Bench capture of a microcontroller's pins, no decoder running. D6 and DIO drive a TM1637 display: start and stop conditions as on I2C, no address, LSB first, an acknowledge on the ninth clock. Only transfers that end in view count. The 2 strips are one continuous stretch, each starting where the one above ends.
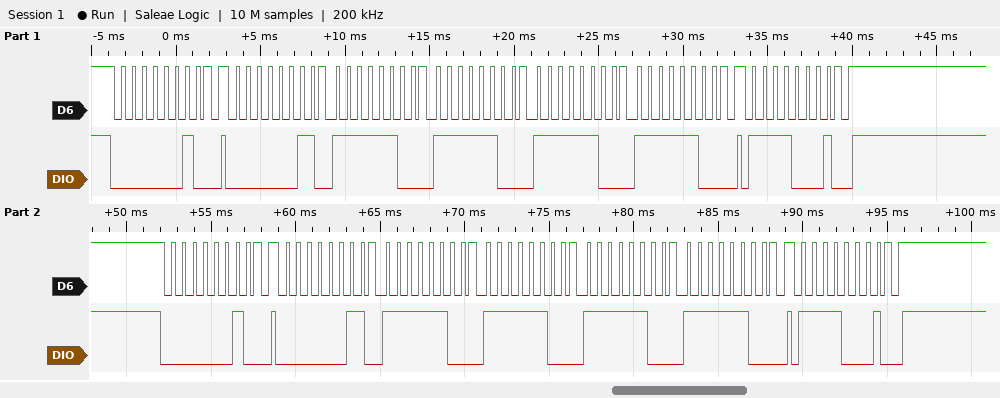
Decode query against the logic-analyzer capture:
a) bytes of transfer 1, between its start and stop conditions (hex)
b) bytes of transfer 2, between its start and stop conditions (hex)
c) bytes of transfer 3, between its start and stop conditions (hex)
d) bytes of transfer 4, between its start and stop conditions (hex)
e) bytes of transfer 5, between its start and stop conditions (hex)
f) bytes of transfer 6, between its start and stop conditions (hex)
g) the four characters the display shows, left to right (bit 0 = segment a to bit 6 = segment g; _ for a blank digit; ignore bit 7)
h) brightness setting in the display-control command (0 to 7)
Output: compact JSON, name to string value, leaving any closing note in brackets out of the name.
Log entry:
{"bytes of transfer 1, between its start and stop conditions": "40", "bytes of transfer 2, between its start and stop conditions": "C0 3F 3F 3F 3F", "bytes of transfer 3, between its start and stop conditions": "8F", "bytes of transfer 4, between its start and stop conditions": "40", "bytes of transfer 5, between its start and stop conditions": "C0 3F 3F 3F 3F", "bytes of transfer 6, between its start and stop conditions": "8F", "the four characters the display shows, left to right": "0000", "brightness setting in the display-control command": "7"}
